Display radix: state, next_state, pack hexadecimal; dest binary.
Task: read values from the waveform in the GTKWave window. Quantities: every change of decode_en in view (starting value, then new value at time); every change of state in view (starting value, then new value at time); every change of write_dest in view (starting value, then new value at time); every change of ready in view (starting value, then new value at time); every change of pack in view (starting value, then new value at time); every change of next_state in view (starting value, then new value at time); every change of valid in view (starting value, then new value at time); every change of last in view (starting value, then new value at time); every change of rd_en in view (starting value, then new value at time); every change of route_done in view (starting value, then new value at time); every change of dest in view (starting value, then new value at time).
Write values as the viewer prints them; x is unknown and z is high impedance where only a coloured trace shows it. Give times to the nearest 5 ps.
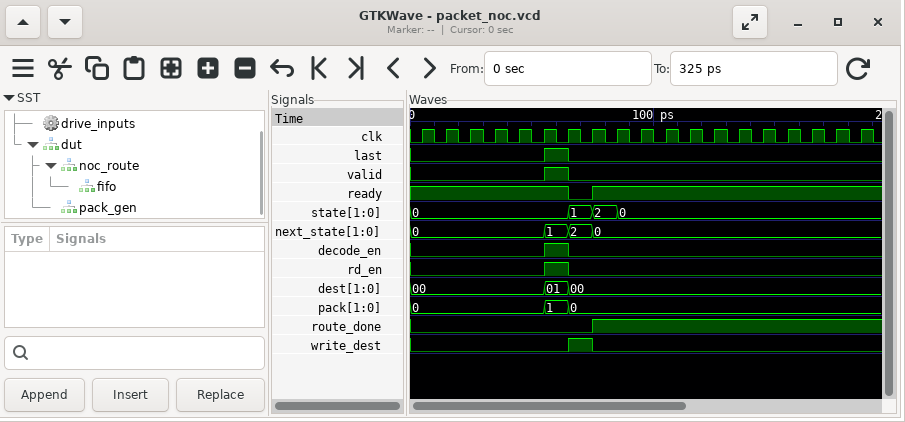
0, 1 at 55 ps, 0 at 65 ps
0, 1 at 65 ps, 2 at 75 ps, 0 at 85 ps
0, 1 at 65 ps, 0 at 75 ps
1, 0 at 65 ps, 1 at 75 ps
0, 1 at 55 ps, 0 at 65 ps
0, 1 at 55 ps, 2 at 65 ps, 0 at 75 ps
0, 1 at 55 ps, 0 at 65 ps
0, 1 at 55 ps, 0 at 65 ps
0, 1 at 55 ps, 0 at 65 ps
0, 1 at 75 ps
00, 01 at 55 ps, 00 at 65 ps
